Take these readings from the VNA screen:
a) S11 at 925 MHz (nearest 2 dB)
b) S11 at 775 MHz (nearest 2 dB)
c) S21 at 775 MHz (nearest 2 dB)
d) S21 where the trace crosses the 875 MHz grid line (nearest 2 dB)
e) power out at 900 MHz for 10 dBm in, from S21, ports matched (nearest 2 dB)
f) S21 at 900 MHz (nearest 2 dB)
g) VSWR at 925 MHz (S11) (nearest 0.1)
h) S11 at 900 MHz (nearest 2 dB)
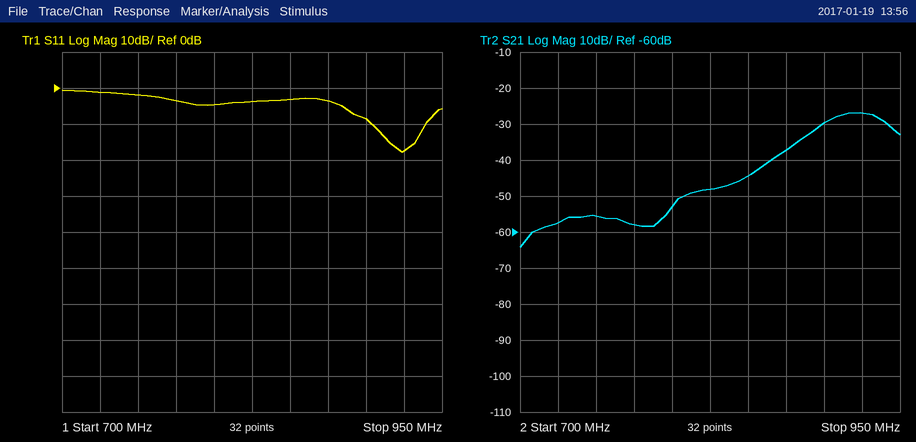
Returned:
-18 dB
-4 dB
-58 dB
-38 dB
-20 dBm
-30 dB
1.3
-8 dB
